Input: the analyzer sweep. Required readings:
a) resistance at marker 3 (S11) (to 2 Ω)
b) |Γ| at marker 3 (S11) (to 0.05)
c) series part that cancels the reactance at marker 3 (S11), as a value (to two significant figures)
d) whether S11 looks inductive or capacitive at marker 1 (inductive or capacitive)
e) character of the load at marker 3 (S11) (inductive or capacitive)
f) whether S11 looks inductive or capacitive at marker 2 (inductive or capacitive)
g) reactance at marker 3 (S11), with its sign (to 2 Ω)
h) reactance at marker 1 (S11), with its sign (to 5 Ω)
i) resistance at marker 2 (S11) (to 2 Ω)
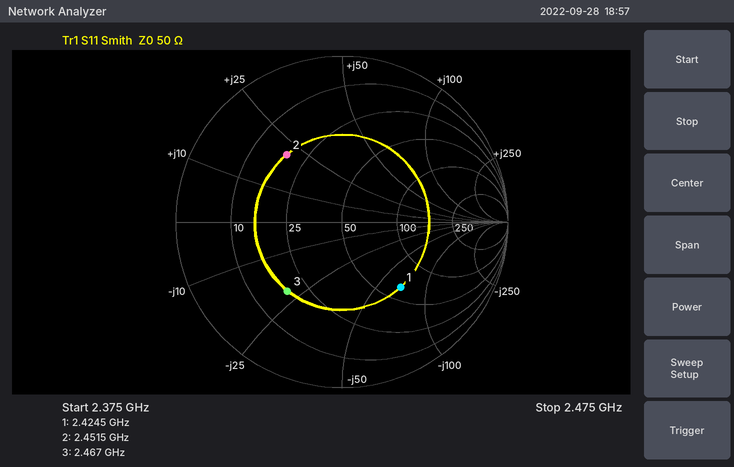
18 Ω
0.55
1.4 nH
capacitive
capacitive
inductive
-22 Ω
-70 Ω
18 Ω
